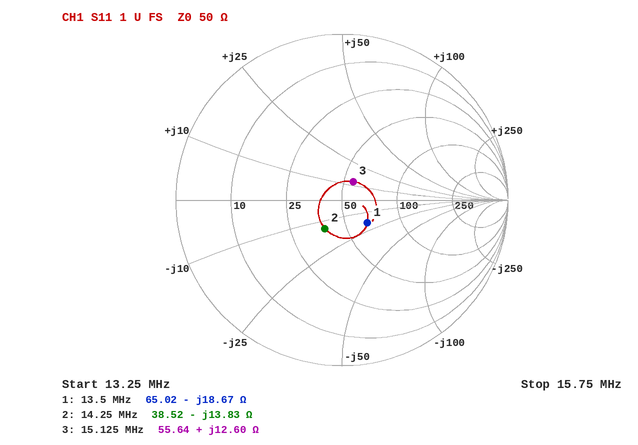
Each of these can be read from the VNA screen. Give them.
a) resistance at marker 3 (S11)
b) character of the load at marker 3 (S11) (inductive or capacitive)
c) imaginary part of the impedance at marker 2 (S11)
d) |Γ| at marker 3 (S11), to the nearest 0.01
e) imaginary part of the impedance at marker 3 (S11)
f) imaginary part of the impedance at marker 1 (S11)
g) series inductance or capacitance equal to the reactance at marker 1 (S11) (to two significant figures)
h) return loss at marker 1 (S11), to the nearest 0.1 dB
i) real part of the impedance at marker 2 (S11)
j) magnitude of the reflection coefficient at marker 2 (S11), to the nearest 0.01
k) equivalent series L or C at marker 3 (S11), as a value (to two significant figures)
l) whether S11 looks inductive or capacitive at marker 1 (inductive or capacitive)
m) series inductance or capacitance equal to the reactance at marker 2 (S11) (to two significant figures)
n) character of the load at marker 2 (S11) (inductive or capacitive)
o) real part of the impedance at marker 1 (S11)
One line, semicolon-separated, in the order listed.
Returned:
55.64 Ω; inductive; -13.83 Ω; 0.13; +12.60 Ω; -18.67 Ω; 630 pF; 13.7 dB; 38.52 Ω; 0.20; 130 nH; capacitive; 810 pF; capacitive; 65.02 Ω
